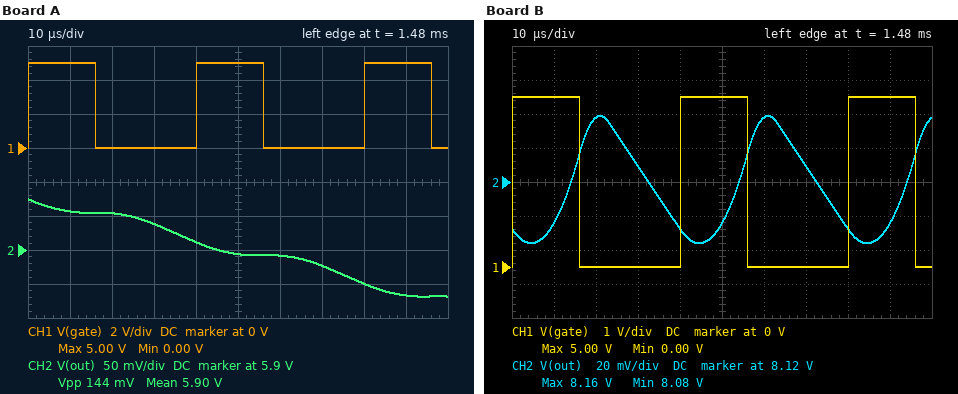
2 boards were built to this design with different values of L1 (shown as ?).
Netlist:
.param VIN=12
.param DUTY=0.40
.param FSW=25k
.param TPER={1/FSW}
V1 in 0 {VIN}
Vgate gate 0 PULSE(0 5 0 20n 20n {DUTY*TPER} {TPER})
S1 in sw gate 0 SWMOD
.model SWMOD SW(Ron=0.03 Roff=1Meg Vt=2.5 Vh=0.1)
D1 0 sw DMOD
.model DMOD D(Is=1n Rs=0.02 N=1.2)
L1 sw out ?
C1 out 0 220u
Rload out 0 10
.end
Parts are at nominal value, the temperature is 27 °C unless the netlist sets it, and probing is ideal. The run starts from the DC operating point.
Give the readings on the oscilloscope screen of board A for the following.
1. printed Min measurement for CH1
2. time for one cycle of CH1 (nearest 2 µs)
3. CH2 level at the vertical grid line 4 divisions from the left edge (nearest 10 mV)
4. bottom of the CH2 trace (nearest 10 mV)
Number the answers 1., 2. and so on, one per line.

1. 0.00 V
2. 40 µs
3. 5.91 V
4. 5.83 V
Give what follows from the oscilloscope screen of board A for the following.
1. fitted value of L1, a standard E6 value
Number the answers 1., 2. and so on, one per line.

1. 150 µH
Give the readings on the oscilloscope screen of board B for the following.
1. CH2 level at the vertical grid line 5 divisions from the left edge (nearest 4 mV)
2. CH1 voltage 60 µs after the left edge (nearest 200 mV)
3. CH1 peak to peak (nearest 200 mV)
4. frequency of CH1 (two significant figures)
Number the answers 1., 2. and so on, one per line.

1. 8.096 V
2. 0 V
3. 5.0 V
4. 25 kHz
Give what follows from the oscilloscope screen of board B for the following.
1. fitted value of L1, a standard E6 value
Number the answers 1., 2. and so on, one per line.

1. 22 µH
